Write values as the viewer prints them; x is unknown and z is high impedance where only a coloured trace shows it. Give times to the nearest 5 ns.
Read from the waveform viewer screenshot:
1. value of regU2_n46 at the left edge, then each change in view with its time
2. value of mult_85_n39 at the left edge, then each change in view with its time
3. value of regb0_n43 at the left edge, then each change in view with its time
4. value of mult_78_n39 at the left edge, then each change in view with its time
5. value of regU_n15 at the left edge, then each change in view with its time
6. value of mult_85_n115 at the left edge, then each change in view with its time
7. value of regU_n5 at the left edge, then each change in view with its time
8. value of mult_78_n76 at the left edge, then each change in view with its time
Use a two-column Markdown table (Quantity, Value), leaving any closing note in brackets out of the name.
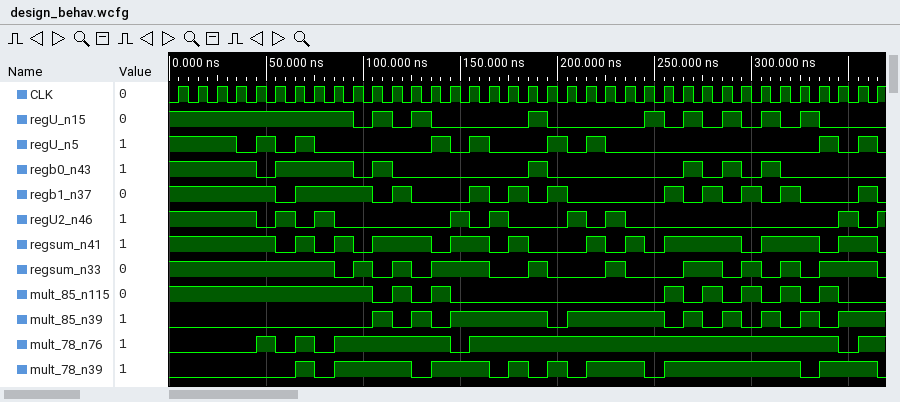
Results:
| Quantity | Value |
|---|---|
| value of regU2_n46 at the left edge, then each change in view with its time | 1, 0 at 45 ns, 1 at 55 ns, 0 at 65 ns, 1 at 75 ns, 0 at 85 ns, 1 at 145 ns, 0 at 155 ns, 1 at 165 ns, 0 at 175 ns, 1 at 205 ns, 0 at 215 ns, 1 at 225 ns, 0 at 235 ns, 1 at 345 ns, 0 at 355 ns, 1 at 365 ns |
| value of mult_85_n39 at the left edge, then each change in view with its time | 0, 1 at 105 ns, 0 at 115 ns, 1 at 125 ns, 0 at 135 ns, 1 at 145 ns, 0 at 195 ns, 1 at 205 ns, 0 at 255 ns, 1 at 265 ns, 0 at 275 ns, 1 at 285 ns, 0 at 295 ns, 1 at 305 ns, 0 at 315 ns, 1 at 325 ns, 0 at 335 ns, 1 at 345 ns |
| value of regb0_n43 at the left edge, then each change in view with its time | 1, 0 at 45 ns, 1 at 55 ns, 0 at 95 ns, 1 at 105 ns, 0 at 115 ns, 1 at 185 ns, 0 at 195 ns, 1 at 265 ns, 0 at 275 ns, 1 at 285 ns, 0 at 295 ns, 1 at 305 ns, 0 at 315 ns |
| value of mult_78_n39 at the left edge, then each change in view with its time | 0, 1 at 65 ns, 0 at 75 ns, 1 at 85 ns, 0 at 125 ns, 1 at 135 ns, 0 at 165 ns, 1 at 175 ns, 0 at 185 ns, 1 at 195 ns, 0 at 205 ns, 1 at 215 ns, 0 at 245 ns, 1 at 255 ns, 0 at 325 ns, 1 at 335 ns, 0 at 365 ns |
| value of regU_n15 at the left edge, then each change in view with its time | 1, 0 at 95 ns, 1 at 105 ns, 0 at 115 ns, 1 at 125 ns, 0 at 135 ns, 1 at 185 ns, 0 at 195 ns, 1 at 245 ns, 0 at 255 ns, 1 at 265 ns, 0 at 275 ns, 1 at 285 ns, 0 at 295 ns, 1 at 305 ns, 0 at 315 ns, 1 at 325 ns, 0 at 335 ns |
| value of mult_85_n115 at the left edge, then each change in view with its time | 1, 0 at 105 ns, 1 at 115 ns, 0 at 125 ns, 1 at 135 ns, 0 at 145 ns, 1 at 255 ns, 0 at 265 ns, 1 at 275 ns, 0 at 285 ns, 1 at 295 ns, 0 at 305 ns, 1 at 315 ns, 0 at 325 ns, 1 at 335 ns, 0 at 345 ns |
| value of regU_n5 at the left edge, then each change in view with its time | 1, 0 at 35 ns, 1 at 45 ns, 0 at 55 ns, 1 at 65 ns, 0 at 75 ns, 1 at 135 ns, 0 at 145 ns, 1 at 155 ns, 0 at 165 ns, 1 at 195 ns, 0 at 205 ns, 1 at 215 ns, 0 at 225 ns, 1 at 335 ns, 0 at 345 ns, 1 at 355 ns, 0 at 365 ns |
| value of mult_78_n76 at the left edge, then each change in view with its time | 0, 1 at 45 ns, 0 at 55 ns, 1 at 65 ns, 0 at 75 ns, 1 at 85 ns, 0 at 145 ns, 1 at 155 ns, 0 at 345 ns, 1 at 355 ns |
